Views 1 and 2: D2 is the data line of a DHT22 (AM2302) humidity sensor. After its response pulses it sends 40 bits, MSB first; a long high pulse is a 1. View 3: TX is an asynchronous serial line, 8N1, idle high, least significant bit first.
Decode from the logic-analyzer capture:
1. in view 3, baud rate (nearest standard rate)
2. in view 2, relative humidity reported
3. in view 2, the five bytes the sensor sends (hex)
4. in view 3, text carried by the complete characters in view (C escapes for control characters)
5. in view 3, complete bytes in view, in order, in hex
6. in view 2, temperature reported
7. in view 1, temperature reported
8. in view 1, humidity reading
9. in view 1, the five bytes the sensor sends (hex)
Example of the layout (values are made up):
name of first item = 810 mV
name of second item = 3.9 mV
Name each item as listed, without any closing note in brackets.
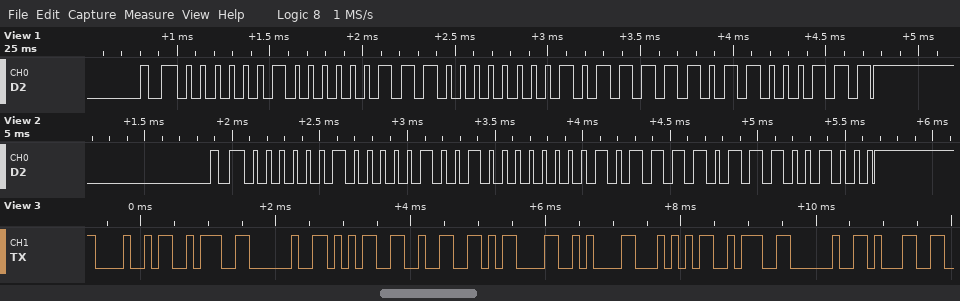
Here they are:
in view 3, baud rate = 9600 baud
in view 2, relative humidity reported = 52.1 %
in view 2, the five bytes the sensor sends = 02 09 00 BD C8
in view 3, text carried by the complete characters in view = "H: 52\r\nT: 1"
in view 3, complete bytes in view, in order, in hex = 48 3A 20 35 32 0D 0A 54 3A 20 31
in view 2, temperature reported = 18.9 °C
in view 1, temperature reported = 19.0 °C
in view 1, humidity reading = 51.9 %
in view 1, the five bytes the sensor sends = 02 07 00 BE C7
